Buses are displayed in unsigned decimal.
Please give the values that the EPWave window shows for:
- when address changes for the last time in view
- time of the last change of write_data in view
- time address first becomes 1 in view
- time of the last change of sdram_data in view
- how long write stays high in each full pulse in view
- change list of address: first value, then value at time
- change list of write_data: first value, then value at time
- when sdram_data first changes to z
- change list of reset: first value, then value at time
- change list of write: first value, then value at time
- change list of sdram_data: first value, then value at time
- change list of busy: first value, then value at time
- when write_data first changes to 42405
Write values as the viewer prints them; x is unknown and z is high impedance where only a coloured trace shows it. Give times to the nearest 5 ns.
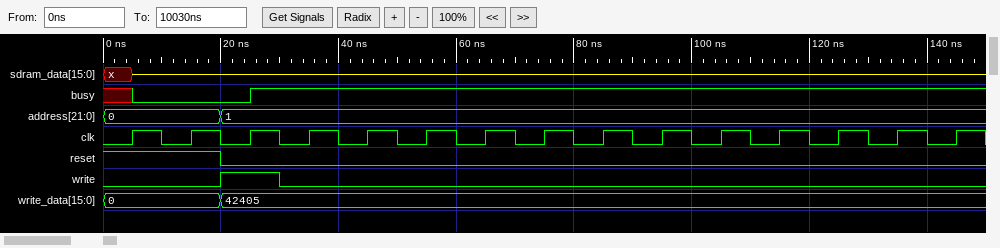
20 ns
20 ns
20 ns
5 ns
10 ns
0, 1 at 20 ns
0, 42405 at 20 ns
5 ns
1, 0 at 20 ns
0, 1 at 20 ns, 0 at 30 ns
x, z at 5 ns
x, 0 at 5 ns, 1 at 25 ns
20 ns
